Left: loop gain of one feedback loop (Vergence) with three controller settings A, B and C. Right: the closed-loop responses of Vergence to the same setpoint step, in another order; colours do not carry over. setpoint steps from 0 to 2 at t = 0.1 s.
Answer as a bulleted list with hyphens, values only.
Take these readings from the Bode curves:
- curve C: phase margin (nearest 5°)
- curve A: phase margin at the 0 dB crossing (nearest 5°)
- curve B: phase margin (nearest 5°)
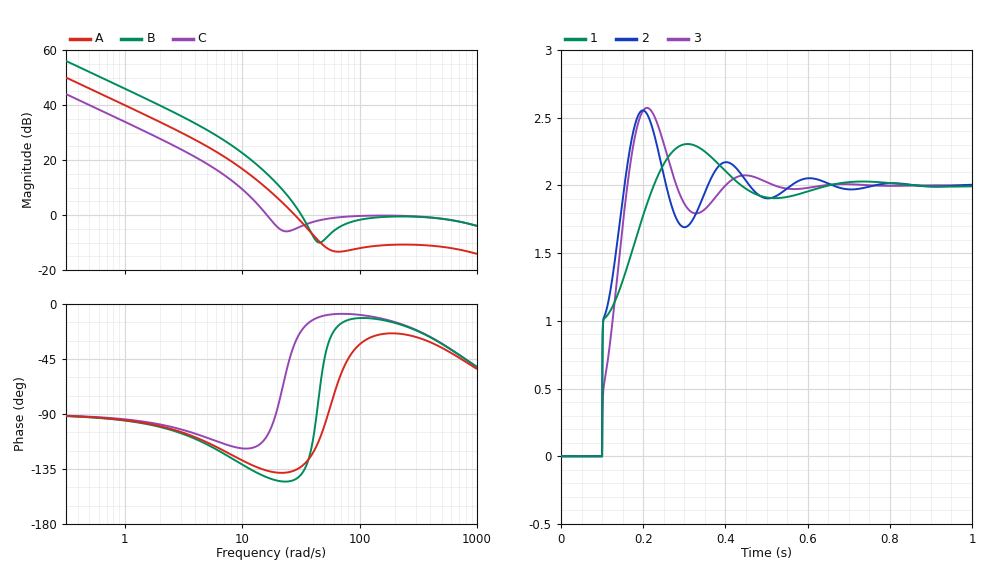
- 70°
- 45°
- 40°
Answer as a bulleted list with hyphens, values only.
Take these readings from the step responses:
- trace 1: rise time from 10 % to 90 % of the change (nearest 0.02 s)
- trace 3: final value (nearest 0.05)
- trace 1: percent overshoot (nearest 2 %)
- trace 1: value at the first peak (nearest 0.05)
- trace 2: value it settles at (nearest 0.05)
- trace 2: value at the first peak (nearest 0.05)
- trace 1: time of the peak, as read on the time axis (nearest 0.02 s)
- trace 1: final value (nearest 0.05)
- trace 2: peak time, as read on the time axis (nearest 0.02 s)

- 0.10 s
- 2.00
- 16 %
- 2.30
- 2.00
- 2.55
- 0.30 s
- 2.00
- 0.20 s
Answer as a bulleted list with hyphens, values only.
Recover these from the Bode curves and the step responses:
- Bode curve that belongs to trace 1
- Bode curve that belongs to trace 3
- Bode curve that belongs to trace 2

- C
- A
- B
